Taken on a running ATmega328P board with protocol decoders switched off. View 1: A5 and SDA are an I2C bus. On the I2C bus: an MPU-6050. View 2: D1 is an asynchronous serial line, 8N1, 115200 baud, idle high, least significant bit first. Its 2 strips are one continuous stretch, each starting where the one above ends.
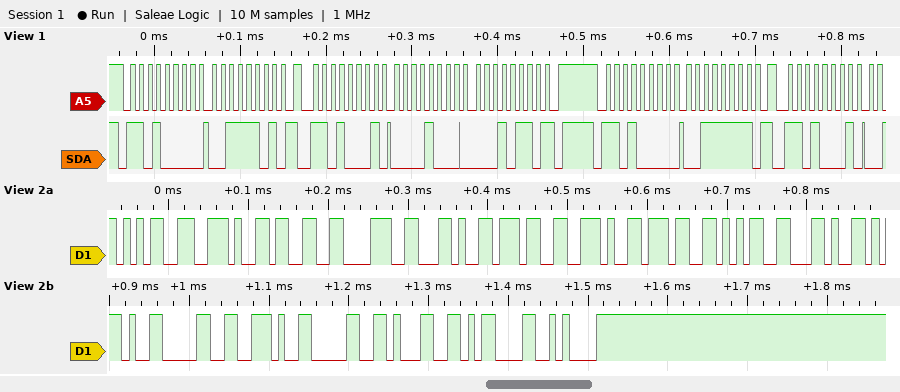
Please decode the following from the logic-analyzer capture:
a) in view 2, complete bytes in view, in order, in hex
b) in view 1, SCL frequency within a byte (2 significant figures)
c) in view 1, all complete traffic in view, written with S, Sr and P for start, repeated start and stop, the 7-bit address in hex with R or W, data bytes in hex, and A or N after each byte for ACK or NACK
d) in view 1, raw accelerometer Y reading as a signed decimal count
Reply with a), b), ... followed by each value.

a) 35 2E 33 38 2C 37 2E 37 35 2C 2D 30 2E 30 31 0D 0A
b) 100 kHz
c) S 68W A 3D A Sr 68R A 08 A 16 N P S 68W A 3F A Sr 68R A
d) 2070
